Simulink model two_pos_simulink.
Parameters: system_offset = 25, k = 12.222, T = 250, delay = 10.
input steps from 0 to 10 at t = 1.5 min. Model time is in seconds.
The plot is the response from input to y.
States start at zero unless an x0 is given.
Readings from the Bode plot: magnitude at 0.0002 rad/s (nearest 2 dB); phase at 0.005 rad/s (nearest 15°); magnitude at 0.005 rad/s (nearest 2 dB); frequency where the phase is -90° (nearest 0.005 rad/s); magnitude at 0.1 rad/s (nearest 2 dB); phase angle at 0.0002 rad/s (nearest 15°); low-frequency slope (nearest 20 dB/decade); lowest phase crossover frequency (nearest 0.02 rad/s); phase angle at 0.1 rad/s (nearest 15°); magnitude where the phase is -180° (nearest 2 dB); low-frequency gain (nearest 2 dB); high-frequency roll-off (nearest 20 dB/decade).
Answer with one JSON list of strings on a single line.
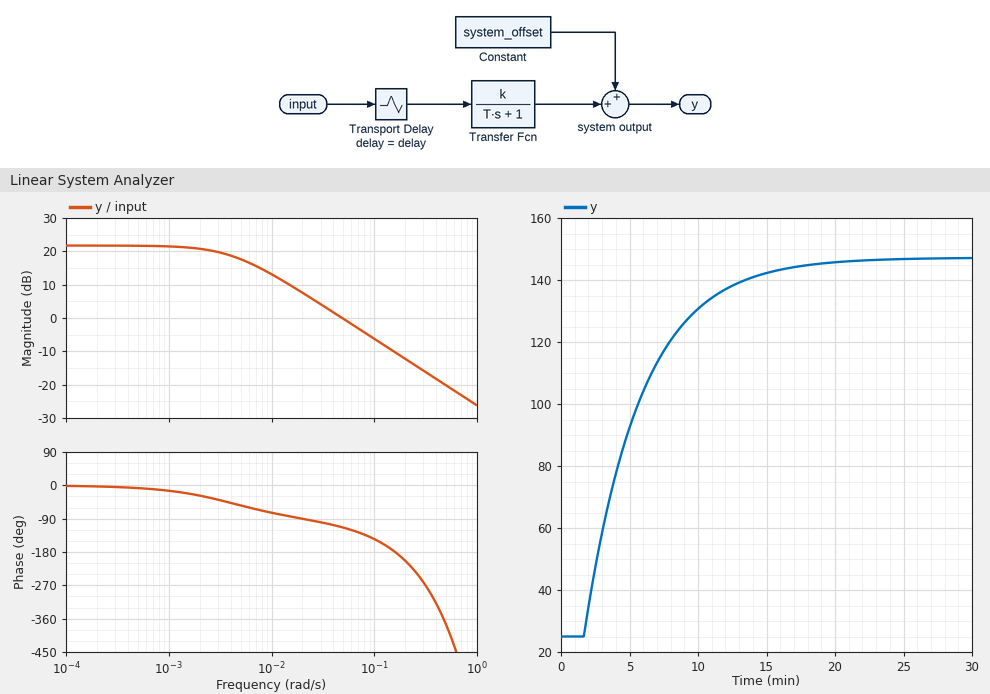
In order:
["22 dB", "-60°", "18 dB", "0.020 rad/s", "-6 dB", "0°", "0 dB/decade", "0.16 rad/s", "-150°", "-10 dB", "22 dB", "-20 dB/decade"]
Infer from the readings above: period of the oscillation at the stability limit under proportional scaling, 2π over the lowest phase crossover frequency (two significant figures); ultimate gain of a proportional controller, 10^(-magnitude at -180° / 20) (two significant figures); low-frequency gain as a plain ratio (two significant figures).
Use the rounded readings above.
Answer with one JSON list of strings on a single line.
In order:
["39 s", "3.2", "13"]
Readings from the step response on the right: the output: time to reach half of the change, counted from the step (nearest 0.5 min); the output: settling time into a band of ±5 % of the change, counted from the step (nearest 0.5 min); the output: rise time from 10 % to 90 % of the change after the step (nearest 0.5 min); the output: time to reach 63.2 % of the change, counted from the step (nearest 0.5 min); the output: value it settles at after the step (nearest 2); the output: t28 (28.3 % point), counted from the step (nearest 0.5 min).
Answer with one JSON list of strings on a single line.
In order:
["3.0 min", "12.5 min", "9.0 min", "4.5 min", "148", "1.5 min"]
